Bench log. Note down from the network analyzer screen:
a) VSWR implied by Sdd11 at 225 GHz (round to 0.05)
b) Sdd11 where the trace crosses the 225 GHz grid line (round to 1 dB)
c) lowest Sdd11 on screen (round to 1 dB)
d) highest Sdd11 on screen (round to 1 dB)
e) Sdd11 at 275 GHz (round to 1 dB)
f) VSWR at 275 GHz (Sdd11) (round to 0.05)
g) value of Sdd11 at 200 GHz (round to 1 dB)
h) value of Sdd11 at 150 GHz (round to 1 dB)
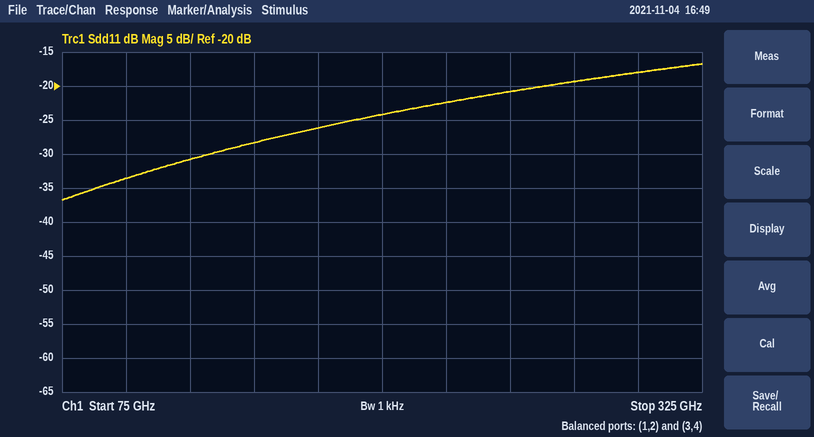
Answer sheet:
1.15
-22 dB
-37 dB
-17 dB
-19 dB
1.25
-24 dB
-28 dB
